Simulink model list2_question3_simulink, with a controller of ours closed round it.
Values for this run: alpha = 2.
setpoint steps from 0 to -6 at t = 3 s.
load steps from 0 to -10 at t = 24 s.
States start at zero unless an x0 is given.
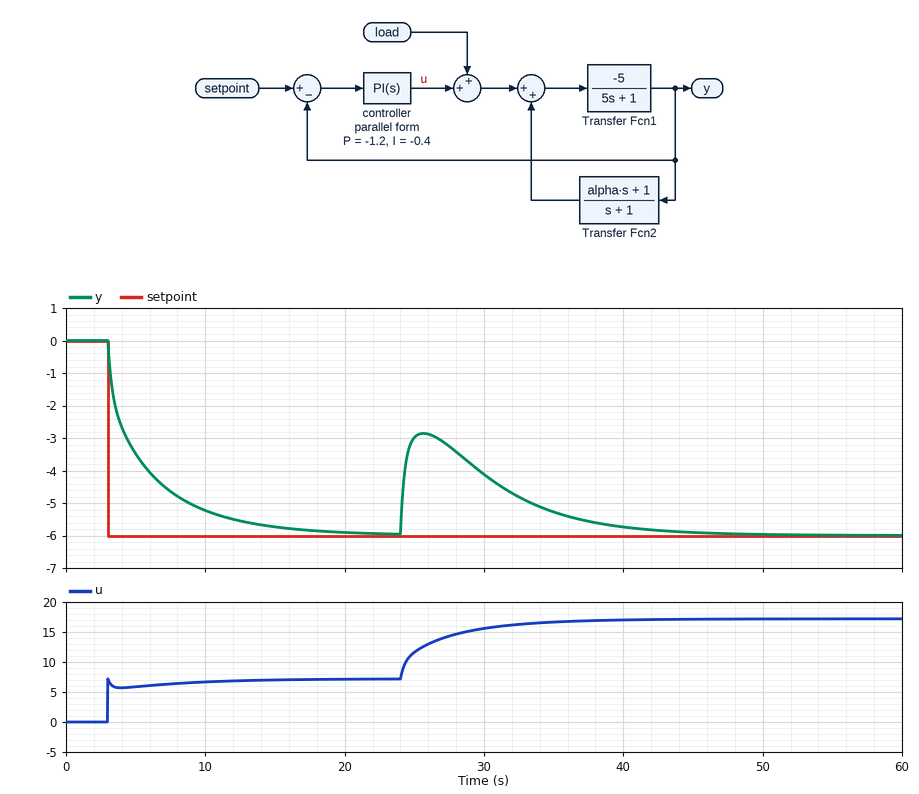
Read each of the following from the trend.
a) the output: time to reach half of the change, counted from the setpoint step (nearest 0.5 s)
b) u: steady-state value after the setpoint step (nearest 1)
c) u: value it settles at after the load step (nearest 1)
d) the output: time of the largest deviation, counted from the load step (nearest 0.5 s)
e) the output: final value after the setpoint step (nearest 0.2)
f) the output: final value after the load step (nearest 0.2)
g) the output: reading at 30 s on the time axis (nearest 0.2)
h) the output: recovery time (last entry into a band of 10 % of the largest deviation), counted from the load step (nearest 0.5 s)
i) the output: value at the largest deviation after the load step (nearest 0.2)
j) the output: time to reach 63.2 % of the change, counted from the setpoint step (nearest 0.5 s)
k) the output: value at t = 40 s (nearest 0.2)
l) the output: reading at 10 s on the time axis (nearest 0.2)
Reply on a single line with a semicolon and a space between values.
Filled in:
1.5 s; 7; 17; 1.5 s; -6.0; -6.0; -4.2; 15.0 s; -2.8; 2.5 s; -5.8; -5.2
